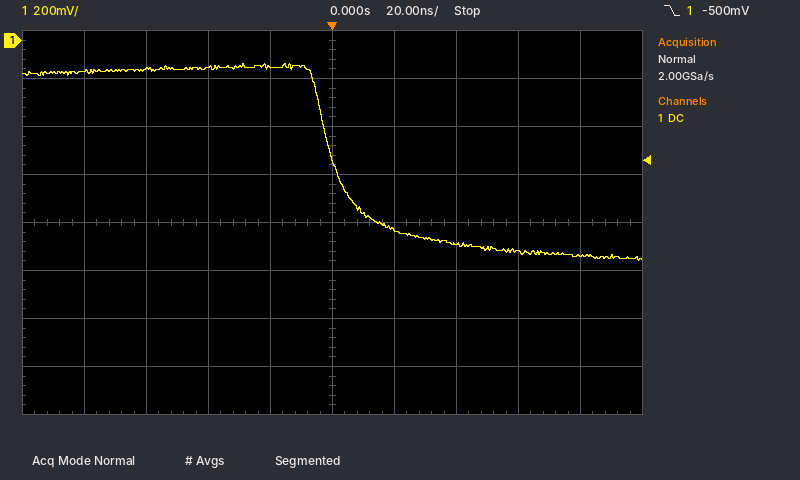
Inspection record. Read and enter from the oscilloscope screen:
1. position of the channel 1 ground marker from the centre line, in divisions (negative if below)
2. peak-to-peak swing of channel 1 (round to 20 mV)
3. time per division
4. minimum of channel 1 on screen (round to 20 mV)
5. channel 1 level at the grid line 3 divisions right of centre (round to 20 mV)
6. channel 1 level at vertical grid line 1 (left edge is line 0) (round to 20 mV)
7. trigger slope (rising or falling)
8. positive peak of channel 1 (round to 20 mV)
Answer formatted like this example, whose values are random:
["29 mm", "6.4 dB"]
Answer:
["+3.8 div", "820 mV", "20 ns", "-920 mV", "-880 mV", "-120 mV", "falling", "-100 mV"]
